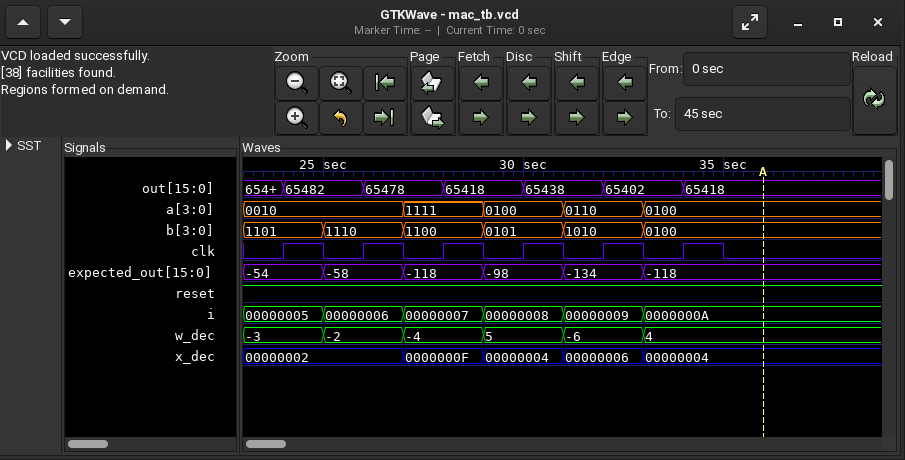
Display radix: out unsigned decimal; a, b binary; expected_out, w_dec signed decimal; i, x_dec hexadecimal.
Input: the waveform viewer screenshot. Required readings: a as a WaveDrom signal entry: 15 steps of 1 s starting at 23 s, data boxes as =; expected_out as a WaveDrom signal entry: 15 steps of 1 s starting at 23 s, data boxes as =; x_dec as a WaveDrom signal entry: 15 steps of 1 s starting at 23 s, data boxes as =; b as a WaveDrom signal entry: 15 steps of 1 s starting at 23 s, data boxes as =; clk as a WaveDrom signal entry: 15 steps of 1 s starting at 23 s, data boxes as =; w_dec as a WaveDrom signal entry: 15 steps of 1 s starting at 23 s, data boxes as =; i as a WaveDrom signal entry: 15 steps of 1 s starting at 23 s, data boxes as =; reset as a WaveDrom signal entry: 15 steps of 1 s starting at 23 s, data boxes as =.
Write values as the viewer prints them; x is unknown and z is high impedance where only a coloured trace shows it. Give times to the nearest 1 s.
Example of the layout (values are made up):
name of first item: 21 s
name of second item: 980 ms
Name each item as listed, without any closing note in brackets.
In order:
a as a WaveDrom signal entry: 15 steps of 1 s starting at 23 s, data boxes as =: {name: 'a', wave: '=...=.=.=.=....', data: '0010 1111 0100 0110 0100'}
expected_out as a WaveDrom signal entry: 15 steps of 1 s starting at 23 s, data boxes as =: {name: 'expected_out', wave: '=.=.=.=.=.=....', data: '-54 -58 -118 -98 -134 -118'}
x_dec as a WaveDrom signal entry: 15 steps of 1 s starting at 23 s, data boxes as =: {name: 'x_dec', wave: '=...=.=.=.=....', data: '00000002 0000000F 00000004 00000006 00000004'}
b as a WaveDrom signal entry: 15 steps of 1 s starting at 23 s, data boxes as =: {name: 'b', wave: '=.=.=.=.=.=....', data: '1101 1110 1100 0101 1010 0100'}
clk as a WaveDrom signal entry: 15 steps of 1 s starting at 23 s, data boxes as =: {name: 'clk', wave: '0101010101010..'}
w_dec as a WaveDrom signal entry: 15 steps of 1 s starting at 23 s, data boxes as =: {name: 'w_dec', wave: '=.=.=.=.=.=....', data: '-3 -2 -4 5 -6 4'}
i as a WaveDrom signal entry: 15 steps of 1 s starting at 23 s, data boxes as =: {name: 'i', wave: '=.=.=.=.=.=....', data: '00000005 00000006 00000007 00000008 00000009 0000000A'}
reset as a WaveDrom signal entry: 15 steps of 1 s starting at 23 s, data boxes as =: {name: 'reset', wave: '1..............'}
